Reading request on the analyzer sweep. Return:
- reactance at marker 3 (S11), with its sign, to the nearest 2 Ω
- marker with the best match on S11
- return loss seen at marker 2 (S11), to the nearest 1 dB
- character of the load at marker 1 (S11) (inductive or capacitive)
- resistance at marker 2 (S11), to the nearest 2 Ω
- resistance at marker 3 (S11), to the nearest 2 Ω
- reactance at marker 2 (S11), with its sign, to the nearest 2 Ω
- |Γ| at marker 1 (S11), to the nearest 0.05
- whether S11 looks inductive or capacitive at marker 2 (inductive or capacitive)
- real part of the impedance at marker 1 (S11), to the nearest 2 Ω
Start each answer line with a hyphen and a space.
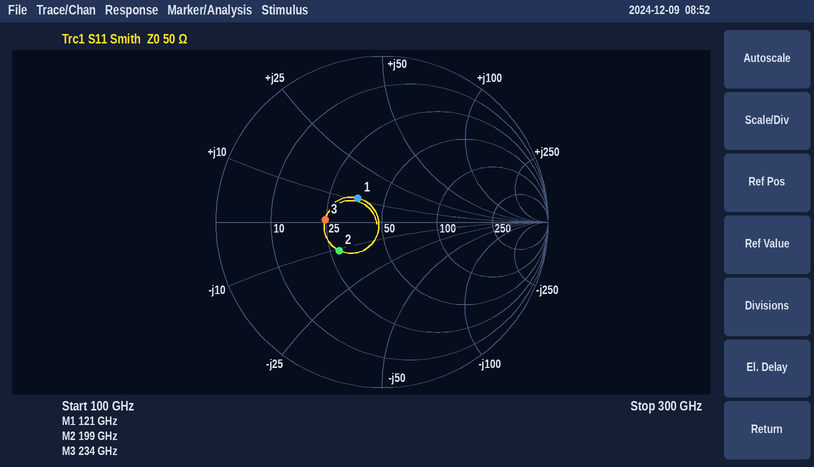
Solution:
- 0 Ω
- marker 1
- 10 dB
- inductive
- 28 Ω
- 24 Ω
- -10 Ω
- 0.20
- capacitive
- 36 Ω
